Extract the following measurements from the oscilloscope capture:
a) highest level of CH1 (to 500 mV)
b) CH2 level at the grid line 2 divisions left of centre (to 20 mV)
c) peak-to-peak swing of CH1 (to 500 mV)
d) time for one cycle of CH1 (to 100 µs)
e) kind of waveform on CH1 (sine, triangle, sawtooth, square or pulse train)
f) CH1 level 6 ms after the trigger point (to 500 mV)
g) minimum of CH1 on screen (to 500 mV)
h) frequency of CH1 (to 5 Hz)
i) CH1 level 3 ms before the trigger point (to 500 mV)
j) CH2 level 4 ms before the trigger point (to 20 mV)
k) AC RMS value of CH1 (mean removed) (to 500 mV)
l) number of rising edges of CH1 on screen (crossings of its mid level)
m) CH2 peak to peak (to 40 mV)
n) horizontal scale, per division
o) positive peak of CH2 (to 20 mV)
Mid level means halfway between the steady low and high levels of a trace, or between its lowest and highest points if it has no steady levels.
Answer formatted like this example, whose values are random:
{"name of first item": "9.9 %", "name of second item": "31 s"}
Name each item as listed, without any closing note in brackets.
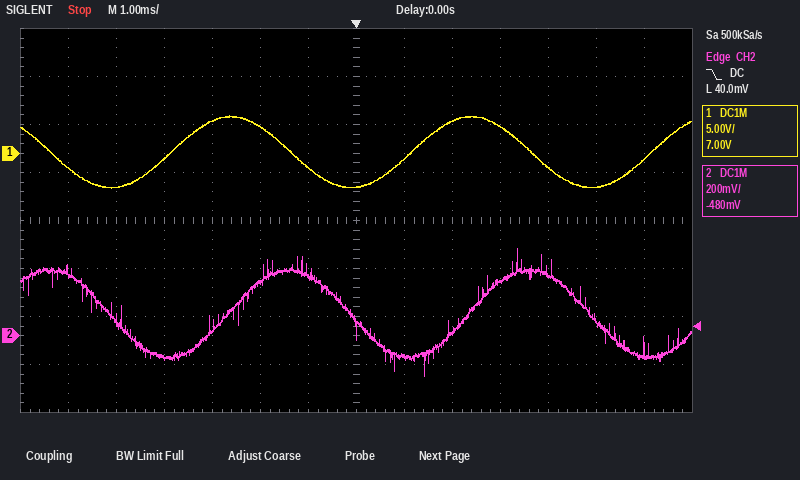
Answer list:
{"highest level of CH1": "4.0 V", "CH2 level at the grid line 2 divisions left of centre": "220 mV", "peak-to-peak swing of CH1": "7.5 V", "time for one cycle of CH1": "5.0 ms", "kind of waveform on CH1": "sine", "CH1 level 6 ms after the trigger point": "-500 mV", "minimum of CH1 on screen": "-3.5 V", "frequency of CH1": "200 Hz", "CH1 level 3 ms before the trigger point": "3.5 V", "CH2 level 4 ms before the trigger point": "-100 mV", "AC RMS value of CH1 (mean removed)": "2.5 V", "number of rising edges of CH1 on screen": "3", "CH2 peak to peak": "520 mV", "horizontal scale, per division": "1 ms", "positive peak of CH2": "360 mV"}
